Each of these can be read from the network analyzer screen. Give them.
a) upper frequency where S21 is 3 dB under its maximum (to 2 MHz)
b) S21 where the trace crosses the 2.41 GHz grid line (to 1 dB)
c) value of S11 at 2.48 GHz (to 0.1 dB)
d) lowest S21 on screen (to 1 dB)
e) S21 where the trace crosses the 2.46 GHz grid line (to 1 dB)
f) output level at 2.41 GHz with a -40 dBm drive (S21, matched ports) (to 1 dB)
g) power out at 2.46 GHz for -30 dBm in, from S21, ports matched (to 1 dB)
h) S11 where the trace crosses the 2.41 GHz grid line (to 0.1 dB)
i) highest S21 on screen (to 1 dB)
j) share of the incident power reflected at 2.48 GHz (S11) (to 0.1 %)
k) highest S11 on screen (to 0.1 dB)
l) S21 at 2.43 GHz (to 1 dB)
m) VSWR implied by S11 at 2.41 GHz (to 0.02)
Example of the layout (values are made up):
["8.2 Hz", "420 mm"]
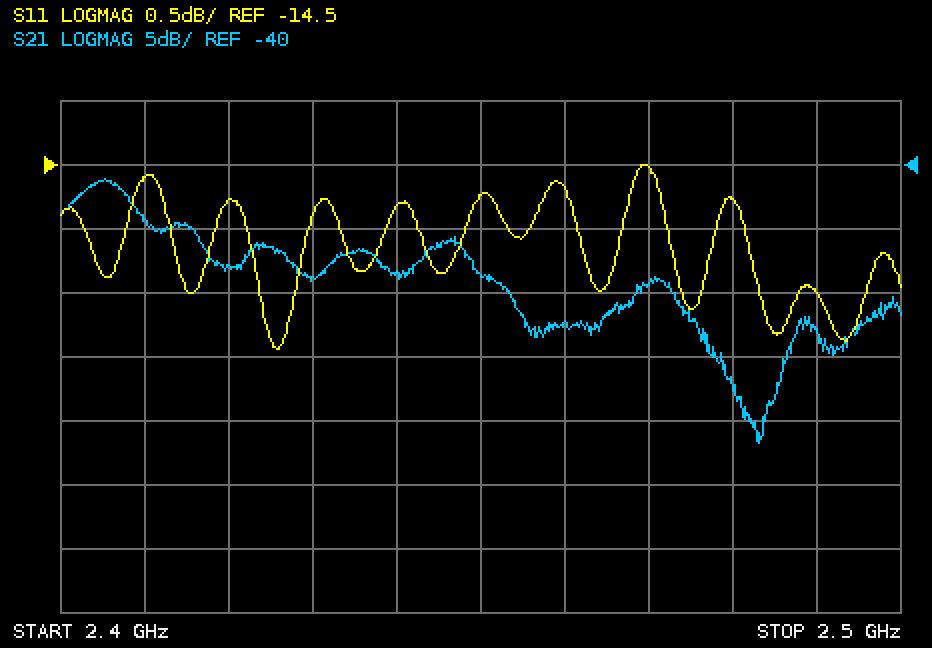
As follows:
["2.410 GHz", "-44 dB", "-14.8 dB", "-62 dB", "-52 dB", "-84 dBm", "-82 dBm", "-14.6 dB", "-41 dB", "3.3 %", "-14.5 dB", "-49 dB", "1.46"]
